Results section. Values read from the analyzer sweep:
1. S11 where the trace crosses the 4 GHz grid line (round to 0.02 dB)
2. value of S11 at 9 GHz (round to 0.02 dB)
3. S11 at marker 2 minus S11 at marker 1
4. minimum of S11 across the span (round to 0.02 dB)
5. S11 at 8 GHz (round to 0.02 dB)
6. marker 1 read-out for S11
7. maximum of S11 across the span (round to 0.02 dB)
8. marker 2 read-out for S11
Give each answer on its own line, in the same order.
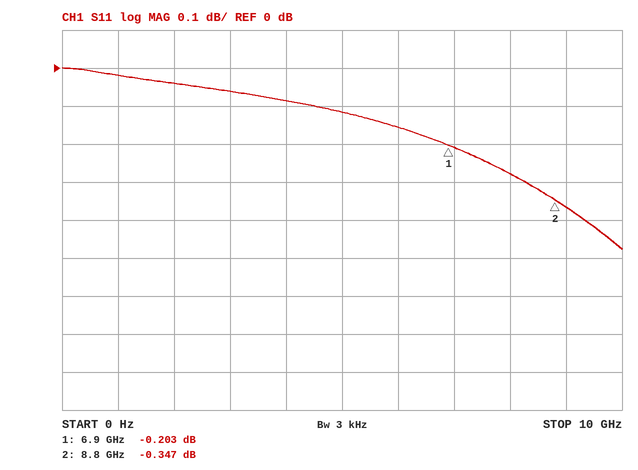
-0.08 dB
-0.36 dB
-0.144 dB
-0.48 dB
-0.28 dB
-0.203 dB
0.00 dB
-0.347 dB
